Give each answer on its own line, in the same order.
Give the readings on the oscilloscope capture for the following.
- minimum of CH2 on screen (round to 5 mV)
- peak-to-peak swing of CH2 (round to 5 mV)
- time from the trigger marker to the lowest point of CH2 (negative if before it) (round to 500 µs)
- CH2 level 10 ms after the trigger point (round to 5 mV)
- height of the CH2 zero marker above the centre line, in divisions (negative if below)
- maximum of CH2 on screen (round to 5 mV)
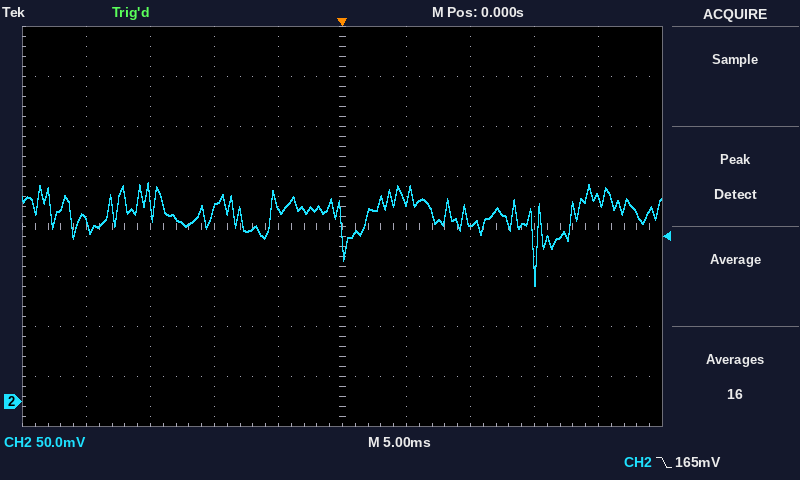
115 mV
105 mV
+15.0 ms
180 mV
-3.5 div
220 mV
